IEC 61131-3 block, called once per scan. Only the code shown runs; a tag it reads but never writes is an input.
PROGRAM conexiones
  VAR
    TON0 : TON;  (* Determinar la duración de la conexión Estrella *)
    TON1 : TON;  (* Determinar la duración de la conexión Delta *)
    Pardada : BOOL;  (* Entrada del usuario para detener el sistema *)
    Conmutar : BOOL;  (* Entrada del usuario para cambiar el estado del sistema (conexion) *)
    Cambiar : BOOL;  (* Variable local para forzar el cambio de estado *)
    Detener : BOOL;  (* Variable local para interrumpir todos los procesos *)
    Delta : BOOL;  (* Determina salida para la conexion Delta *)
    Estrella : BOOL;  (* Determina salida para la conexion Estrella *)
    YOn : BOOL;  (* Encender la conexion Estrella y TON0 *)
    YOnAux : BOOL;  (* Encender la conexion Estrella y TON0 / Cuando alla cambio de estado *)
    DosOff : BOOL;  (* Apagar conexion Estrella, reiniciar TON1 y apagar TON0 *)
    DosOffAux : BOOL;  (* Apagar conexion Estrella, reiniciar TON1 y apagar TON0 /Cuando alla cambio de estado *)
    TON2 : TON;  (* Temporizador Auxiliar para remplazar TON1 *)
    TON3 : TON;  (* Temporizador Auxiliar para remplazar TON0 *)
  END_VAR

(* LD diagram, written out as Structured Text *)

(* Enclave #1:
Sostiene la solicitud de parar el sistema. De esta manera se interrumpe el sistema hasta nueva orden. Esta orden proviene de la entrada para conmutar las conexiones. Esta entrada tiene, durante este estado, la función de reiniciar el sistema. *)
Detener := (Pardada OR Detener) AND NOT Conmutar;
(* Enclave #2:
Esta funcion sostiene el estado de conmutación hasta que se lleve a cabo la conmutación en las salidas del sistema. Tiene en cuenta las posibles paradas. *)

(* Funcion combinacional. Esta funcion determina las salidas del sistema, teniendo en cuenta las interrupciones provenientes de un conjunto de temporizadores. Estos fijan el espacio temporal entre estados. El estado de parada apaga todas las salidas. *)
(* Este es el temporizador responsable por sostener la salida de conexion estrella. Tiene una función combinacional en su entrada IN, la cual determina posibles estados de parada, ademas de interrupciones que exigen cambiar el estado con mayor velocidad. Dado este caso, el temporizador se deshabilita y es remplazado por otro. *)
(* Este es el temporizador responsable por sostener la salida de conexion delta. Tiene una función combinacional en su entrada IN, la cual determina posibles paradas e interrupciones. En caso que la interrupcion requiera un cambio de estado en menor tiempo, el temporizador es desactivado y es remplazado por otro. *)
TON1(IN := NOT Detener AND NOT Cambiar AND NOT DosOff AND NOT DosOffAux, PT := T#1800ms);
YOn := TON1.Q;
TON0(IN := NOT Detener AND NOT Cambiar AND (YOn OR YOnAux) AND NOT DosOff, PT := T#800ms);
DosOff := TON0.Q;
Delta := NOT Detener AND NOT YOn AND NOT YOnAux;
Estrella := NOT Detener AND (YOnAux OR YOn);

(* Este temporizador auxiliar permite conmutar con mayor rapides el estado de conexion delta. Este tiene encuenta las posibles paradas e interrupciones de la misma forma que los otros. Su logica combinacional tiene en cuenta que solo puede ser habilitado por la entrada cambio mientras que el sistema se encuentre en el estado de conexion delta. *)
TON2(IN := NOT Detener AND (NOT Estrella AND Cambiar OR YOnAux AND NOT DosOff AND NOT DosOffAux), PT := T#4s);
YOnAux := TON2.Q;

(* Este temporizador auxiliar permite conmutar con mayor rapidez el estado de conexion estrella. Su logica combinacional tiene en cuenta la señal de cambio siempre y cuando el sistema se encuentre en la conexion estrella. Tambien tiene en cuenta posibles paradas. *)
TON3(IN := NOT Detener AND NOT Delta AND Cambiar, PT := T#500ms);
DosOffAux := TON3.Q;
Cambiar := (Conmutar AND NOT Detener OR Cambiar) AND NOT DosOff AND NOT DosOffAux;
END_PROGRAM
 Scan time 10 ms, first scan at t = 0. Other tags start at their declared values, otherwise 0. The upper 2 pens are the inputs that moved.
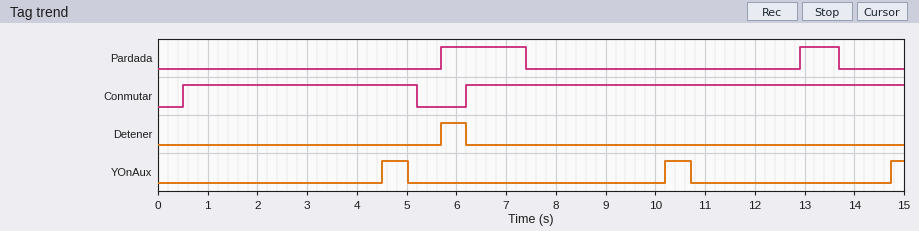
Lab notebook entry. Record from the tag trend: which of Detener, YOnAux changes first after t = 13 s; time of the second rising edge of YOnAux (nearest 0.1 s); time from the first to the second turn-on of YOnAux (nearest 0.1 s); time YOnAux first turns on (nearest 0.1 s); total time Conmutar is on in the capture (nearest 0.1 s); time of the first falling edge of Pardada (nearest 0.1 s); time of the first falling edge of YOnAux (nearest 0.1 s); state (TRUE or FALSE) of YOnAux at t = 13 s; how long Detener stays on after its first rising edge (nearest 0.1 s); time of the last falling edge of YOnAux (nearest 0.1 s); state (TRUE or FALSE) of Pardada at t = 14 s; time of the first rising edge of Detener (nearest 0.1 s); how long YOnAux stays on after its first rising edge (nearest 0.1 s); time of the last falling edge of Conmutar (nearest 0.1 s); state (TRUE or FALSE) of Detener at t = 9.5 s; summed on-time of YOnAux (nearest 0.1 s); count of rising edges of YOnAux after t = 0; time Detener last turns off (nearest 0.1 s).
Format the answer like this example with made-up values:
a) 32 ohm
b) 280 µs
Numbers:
a) YOnAux
b) 10.2 s
c) 5.7 s
d) 4.5 s
e) 13.5 s
f) 7.4 s
g) 5.0 s
h) FALSE
i) 0.5 s
j) 10.7 s
k) FALSE
l) 5.7 s
m) 0.5 s
n) 5.2 s
o) FALSE
p) 1.3 s
q) 3
r) 6.2 s
